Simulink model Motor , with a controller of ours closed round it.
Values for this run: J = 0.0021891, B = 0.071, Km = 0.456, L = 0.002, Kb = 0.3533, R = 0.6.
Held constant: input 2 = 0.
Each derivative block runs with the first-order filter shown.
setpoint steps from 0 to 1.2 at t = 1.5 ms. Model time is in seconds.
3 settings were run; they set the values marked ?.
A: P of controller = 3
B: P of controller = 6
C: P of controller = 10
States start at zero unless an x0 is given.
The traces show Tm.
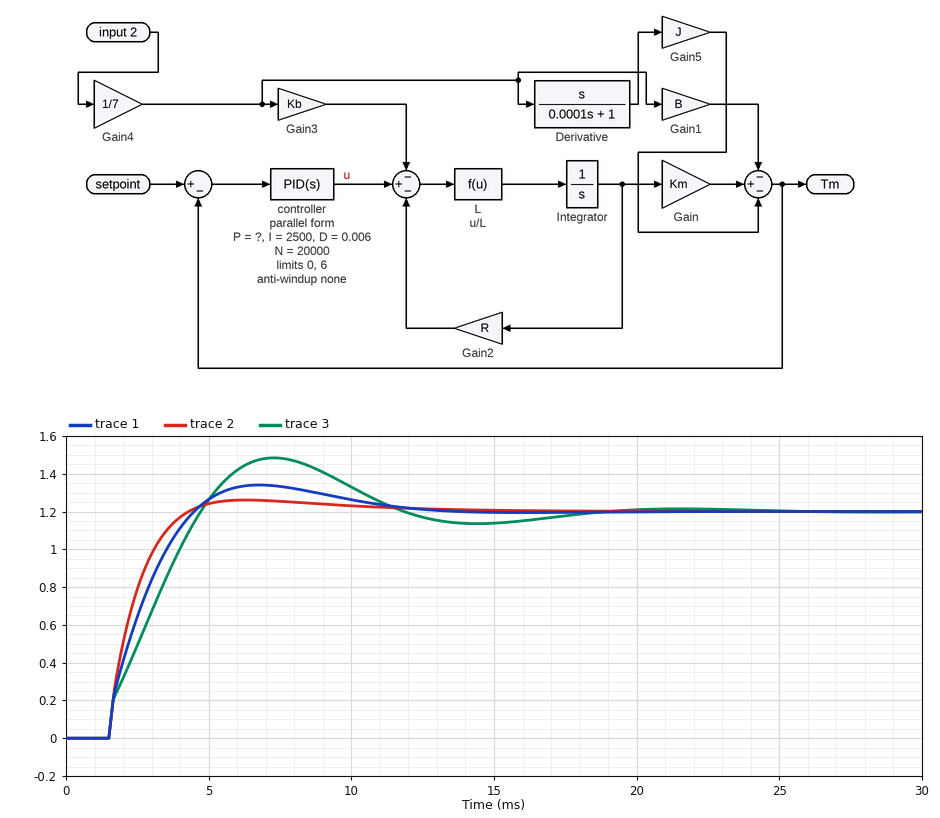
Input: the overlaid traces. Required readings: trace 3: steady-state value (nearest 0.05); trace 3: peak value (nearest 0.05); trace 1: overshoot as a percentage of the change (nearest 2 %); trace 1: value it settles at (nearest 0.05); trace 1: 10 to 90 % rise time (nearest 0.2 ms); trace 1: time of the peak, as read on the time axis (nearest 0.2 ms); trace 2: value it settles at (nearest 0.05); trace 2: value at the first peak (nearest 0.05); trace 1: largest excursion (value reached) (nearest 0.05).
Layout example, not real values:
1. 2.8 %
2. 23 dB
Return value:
1. 1.20
2. 1.50
3. 12 %
4. 1.20
5. 2.2 ms
6. 6.8 ms
7. 1.20
8. 1.25
9. 1.35
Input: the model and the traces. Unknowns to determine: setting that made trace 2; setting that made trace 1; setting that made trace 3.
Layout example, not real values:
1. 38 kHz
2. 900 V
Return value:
1. C
2. B
3. A
